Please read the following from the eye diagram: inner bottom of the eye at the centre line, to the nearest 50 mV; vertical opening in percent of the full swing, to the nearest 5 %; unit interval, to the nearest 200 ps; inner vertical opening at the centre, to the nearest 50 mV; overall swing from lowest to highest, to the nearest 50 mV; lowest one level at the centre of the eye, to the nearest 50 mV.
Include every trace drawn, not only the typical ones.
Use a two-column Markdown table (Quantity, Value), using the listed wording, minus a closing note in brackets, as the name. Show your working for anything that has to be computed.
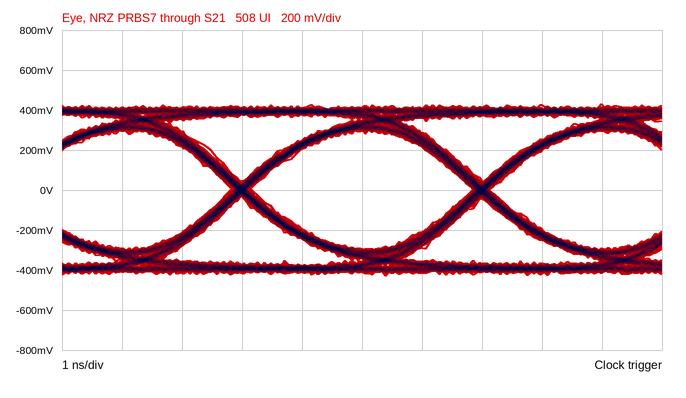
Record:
| Quantity | Value |
|---|---|
| inner bottom of the eye at the centre line, to the nearest 50 mV | -300 mV |
| vertical opening in percent of the full swing, to the nearest 5 % | 600 mV / 850 mV ≈ 70.6 %, so 70 % to the nearest 5 % |
| unit interval, to the nearest 200 ps | 4.0 ns |
| inner vertical opening at the centre, to the nearest 50 mV | 600 mV |
| overall swing from lowest to highest, to the nearest 50 mV | 850 mV |
| lowest one level at the centre of the eye, to the nearest 50 mV | 300 mV |
